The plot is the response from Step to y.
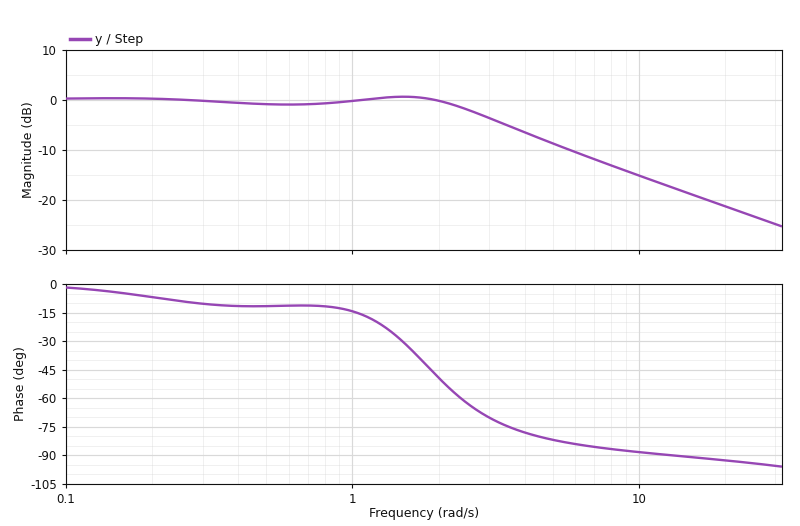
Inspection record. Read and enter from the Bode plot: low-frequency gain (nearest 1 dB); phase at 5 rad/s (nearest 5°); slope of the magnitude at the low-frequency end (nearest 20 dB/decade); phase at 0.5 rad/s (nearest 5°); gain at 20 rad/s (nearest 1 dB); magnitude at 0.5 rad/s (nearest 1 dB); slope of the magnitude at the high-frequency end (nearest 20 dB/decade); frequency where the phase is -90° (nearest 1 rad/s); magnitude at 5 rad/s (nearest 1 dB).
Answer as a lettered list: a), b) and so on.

a) 0 dB
b) -80°
c) 0 dB/decade
d) -10°
e) -21 dB
f) -1 dB
g) -20 dB/decade
h) 13 rad/s
i) -9 dB
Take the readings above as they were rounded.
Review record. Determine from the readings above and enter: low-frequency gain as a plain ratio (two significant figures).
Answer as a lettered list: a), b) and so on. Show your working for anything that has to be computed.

a) 10^(0 / 20) = 1.0
